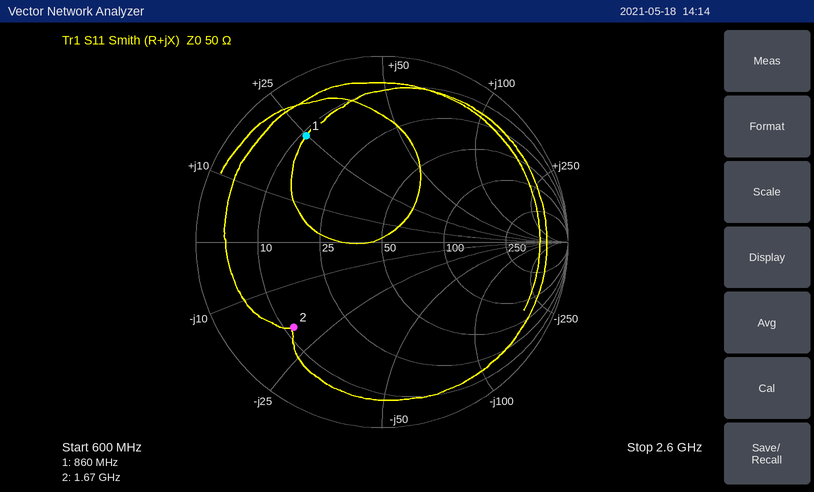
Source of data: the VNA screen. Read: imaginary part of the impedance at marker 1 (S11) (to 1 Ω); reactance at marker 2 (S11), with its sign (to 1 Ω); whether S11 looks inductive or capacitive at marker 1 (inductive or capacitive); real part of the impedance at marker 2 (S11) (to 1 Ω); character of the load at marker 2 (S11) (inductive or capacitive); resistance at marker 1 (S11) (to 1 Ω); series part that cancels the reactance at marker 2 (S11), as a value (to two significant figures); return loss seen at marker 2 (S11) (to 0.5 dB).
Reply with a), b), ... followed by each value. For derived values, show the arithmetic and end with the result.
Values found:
a) +25 Ω
b) -19 Ω
c) inductive
d) 12 Ω
e) capacitive
f) 11 Ω
g) L = 19 Ω/(2π × 1.67 GHz) ≈ 1.8 nH
h) 3.5 dB
